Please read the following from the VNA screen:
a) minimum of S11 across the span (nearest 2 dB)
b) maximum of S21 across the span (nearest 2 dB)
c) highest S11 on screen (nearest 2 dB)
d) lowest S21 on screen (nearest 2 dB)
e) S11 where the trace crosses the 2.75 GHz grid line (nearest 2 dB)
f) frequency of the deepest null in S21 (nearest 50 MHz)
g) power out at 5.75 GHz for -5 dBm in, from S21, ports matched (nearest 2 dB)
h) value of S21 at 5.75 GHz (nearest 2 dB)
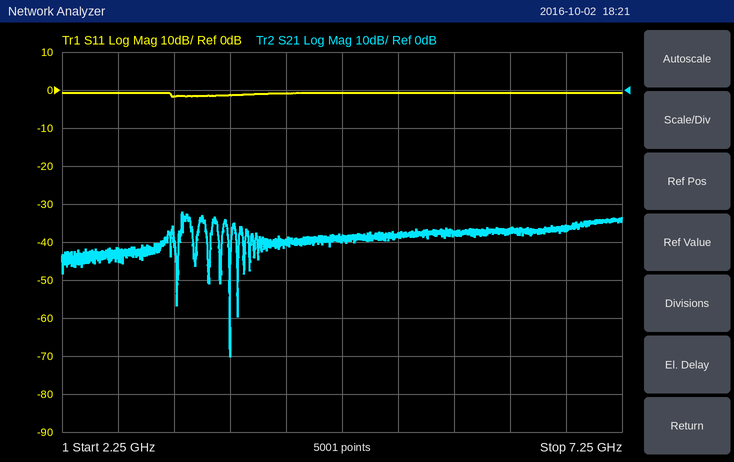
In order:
-2 dB
-32 dB
0 dB
-70 dB
0 dB
3.75 GHz
-42 dBm
-38 dB
